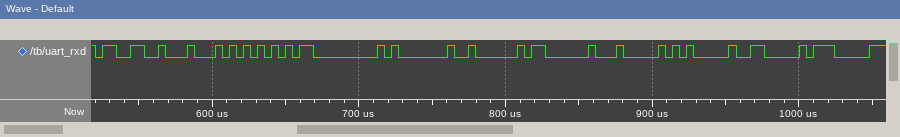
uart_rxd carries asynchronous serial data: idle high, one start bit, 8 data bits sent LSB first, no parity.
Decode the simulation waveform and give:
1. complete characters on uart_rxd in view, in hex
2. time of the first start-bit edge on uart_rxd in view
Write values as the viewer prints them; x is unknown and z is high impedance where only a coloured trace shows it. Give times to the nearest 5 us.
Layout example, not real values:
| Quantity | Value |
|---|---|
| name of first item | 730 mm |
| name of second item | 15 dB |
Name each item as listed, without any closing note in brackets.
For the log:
| Quantity | Value |
|---|---|
| complete characters on uart_rxd in view, in hex | 33, 44, 55, 00, 01, 02, 03, 04, 05, 06, 07 |
| time of the first start-bit edge on uart_rxd in view | 520 us |
